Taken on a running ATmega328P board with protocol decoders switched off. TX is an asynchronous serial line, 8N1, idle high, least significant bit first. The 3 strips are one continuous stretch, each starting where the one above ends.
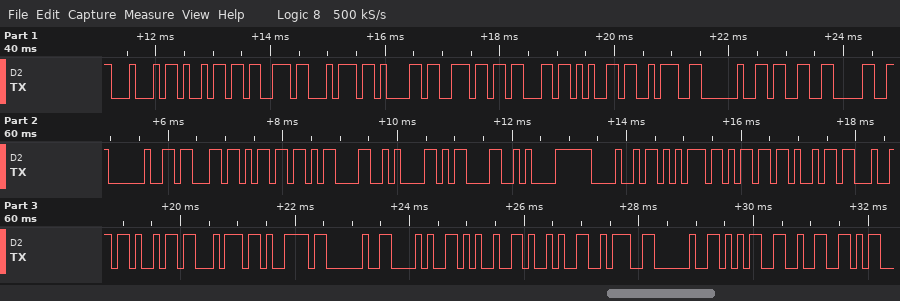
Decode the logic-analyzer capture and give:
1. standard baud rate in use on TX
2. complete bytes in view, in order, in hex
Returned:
9600 baud
0x44 0x69 0x73 0x74 0x61 0x6E 0x63 0x65 0x3A 0x20 0x33 0x30 0x20 0x63 0x6D 0x0D 0x0A 0x0D 0x0A 0x48 0x75 0x6D 0x69 0x64 0x69 0x74 0x79 0x20 0x28 0x25 0x29 0x3A 0x20 0x35 0x32
